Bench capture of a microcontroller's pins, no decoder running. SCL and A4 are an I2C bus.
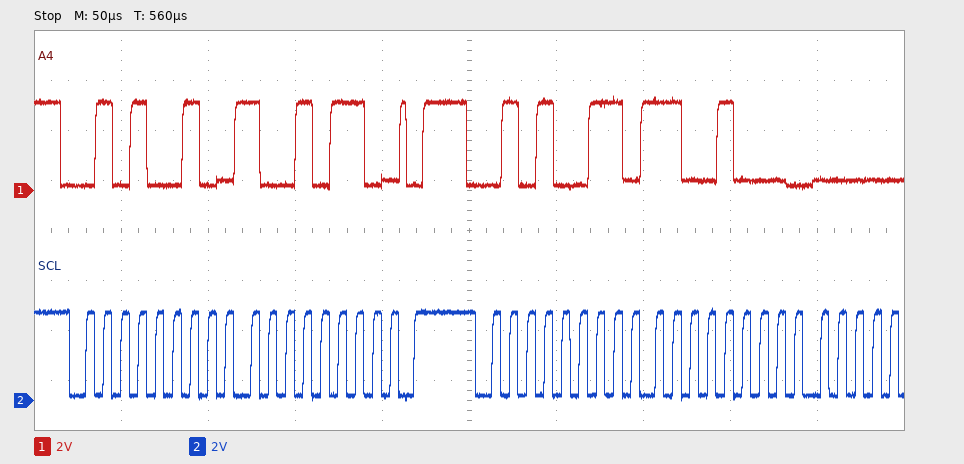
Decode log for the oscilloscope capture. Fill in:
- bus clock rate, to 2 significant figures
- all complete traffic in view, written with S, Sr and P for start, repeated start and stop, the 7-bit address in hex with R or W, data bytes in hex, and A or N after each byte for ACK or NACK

100 kHz
S 29W A 96 A P S 29R A C8 A
